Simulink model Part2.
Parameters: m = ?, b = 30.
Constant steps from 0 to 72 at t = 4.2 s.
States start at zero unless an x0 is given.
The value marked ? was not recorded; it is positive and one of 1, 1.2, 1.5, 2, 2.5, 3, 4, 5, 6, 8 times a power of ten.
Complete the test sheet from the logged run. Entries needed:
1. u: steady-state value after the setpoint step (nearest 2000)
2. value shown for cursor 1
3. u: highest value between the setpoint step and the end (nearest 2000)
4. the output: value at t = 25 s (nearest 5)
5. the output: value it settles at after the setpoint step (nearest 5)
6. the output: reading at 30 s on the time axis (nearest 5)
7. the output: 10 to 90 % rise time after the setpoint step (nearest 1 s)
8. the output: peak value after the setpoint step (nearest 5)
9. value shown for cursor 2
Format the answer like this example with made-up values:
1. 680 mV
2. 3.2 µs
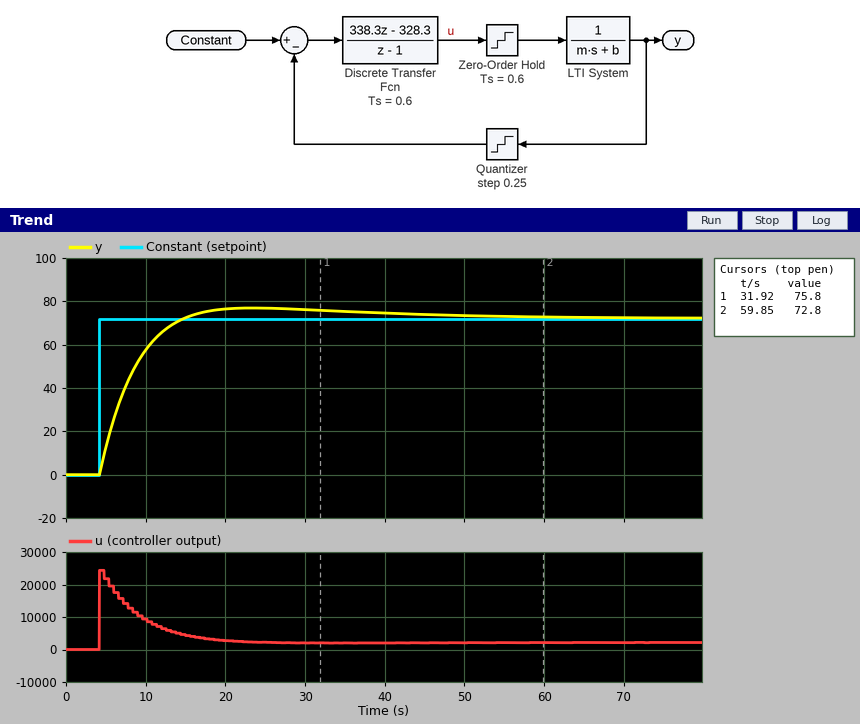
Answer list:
1. 2000
2. 75.8
3. 24000
4. 75
5. 70
6. 75
7. 7 s
8. 75
9. 72.8
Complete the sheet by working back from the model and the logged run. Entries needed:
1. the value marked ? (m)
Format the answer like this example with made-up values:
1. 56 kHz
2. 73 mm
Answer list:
1. 1500
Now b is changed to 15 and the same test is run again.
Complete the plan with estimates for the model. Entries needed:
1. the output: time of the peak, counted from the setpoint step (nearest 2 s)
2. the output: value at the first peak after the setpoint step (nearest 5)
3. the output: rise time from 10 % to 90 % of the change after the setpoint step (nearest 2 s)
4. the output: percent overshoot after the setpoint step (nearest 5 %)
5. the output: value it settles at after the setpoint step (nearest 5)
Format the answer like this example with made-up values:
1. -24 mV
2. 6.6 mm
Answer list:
1. 18 s
2. 80
3. 6 s
4. 10 %
5. 70
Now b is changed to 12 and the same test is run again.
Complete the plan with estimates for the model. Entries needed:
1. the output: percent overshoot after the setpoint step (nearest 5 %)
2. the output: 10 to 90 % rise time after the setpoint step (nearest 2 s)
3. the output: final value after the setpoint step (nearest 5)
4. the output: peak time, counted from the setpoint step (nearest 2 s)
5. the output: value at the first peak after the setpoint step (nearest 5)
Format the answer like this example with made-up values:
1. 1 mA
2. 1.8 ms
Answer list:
1. 10 %
2. 6 s
3. 70
4. 18 s
5. 80
